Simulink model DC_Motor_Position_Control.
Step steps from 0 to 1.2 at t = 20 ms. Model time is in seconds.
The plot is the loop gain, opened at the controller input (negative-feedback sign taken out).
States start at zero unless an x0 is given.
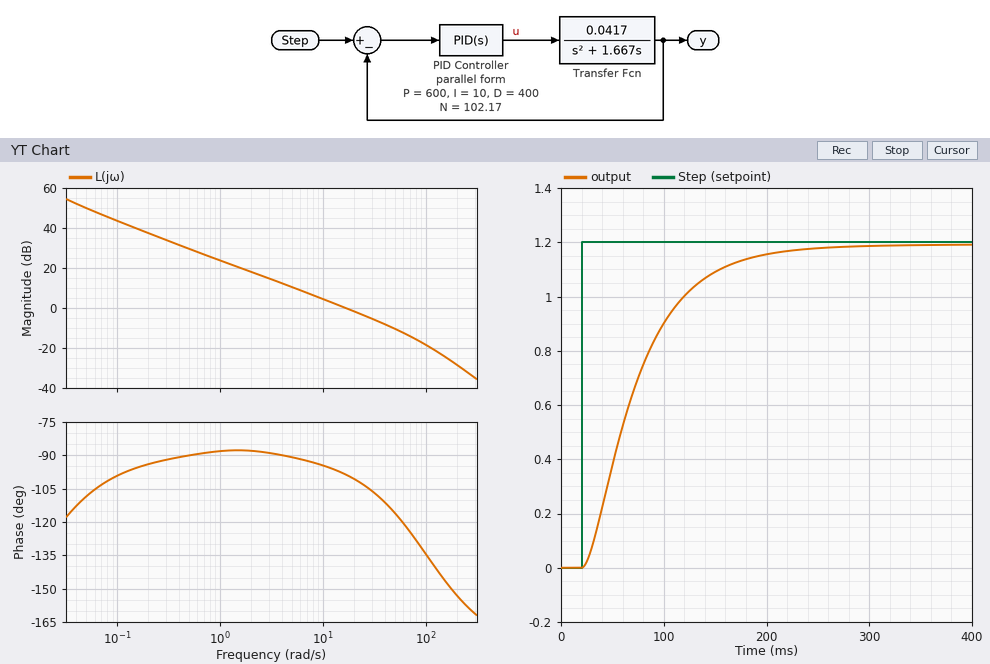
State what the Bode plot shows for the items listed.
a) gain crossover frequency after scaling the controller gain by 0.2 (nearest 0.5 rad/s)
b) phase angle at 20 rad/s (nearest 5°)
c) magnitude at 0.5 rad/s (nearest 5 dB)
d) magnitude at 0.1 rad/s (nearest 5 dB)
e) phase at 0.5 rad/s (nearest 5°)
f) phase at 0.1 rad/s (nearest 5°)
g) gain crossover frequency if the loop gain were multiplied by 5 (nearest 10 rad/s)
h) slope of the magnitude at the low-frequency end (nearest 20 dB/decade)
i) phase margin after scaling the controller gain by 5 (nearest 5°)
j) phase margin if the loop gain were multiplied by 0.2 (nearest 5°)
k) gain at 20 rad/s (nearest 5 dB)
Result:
3.5 rad/s
-100°
30 dB
45 dB
-90°
-100°
70 rad/s
-20 dB/decade
55°
90°
0 dB
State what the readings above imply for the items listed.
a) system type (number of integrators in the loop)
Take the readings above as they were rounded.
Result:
1
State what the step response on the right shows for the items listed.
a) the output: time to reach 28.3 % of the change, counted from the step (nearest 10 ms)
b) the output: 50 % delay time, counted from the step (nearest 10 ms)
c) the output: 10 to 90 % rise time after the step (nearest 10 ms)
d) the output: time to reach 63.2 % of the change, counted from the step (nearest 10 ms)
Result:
30 ms
50 ms
110 ms
60 ms
